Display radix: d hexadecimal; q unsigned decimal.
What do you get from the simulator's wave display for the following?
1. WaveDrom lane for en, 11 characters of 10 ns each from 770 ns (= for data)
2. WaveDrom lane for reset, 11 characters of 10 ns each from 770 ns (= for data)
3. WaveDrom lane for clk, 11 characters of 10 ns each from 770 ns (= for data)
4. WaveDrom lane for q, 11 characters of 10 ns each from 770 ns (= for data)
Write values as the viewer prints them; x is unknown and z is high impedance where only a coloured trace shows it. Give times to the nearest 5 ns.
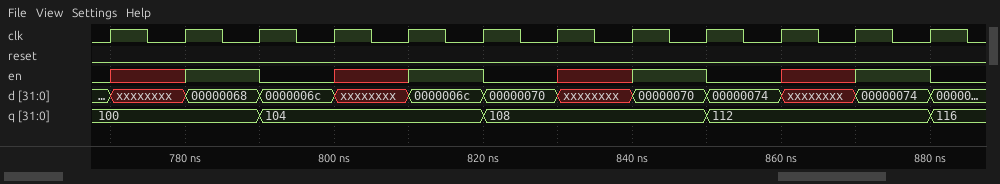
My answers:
{name: 'en', wave: 'x10x10x10x1'}
{name: 'reset', wave: '0..........'}
{name: 'clk', wave: 'p..........'}
{name: 'q', wave: '=.=..=..=..', data: '100 104 108 112'}
